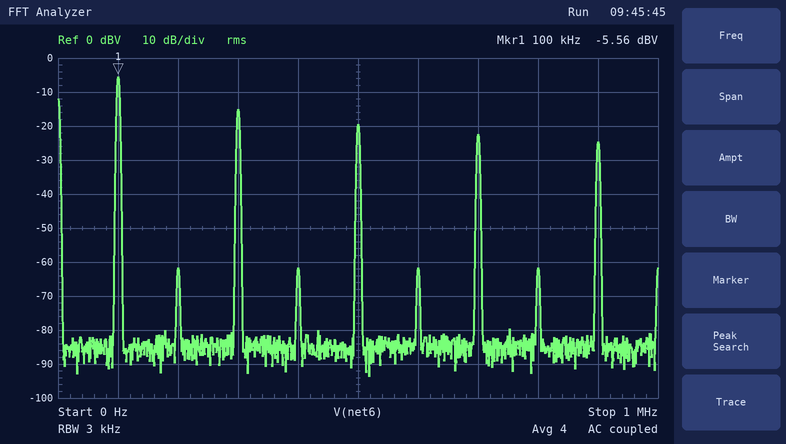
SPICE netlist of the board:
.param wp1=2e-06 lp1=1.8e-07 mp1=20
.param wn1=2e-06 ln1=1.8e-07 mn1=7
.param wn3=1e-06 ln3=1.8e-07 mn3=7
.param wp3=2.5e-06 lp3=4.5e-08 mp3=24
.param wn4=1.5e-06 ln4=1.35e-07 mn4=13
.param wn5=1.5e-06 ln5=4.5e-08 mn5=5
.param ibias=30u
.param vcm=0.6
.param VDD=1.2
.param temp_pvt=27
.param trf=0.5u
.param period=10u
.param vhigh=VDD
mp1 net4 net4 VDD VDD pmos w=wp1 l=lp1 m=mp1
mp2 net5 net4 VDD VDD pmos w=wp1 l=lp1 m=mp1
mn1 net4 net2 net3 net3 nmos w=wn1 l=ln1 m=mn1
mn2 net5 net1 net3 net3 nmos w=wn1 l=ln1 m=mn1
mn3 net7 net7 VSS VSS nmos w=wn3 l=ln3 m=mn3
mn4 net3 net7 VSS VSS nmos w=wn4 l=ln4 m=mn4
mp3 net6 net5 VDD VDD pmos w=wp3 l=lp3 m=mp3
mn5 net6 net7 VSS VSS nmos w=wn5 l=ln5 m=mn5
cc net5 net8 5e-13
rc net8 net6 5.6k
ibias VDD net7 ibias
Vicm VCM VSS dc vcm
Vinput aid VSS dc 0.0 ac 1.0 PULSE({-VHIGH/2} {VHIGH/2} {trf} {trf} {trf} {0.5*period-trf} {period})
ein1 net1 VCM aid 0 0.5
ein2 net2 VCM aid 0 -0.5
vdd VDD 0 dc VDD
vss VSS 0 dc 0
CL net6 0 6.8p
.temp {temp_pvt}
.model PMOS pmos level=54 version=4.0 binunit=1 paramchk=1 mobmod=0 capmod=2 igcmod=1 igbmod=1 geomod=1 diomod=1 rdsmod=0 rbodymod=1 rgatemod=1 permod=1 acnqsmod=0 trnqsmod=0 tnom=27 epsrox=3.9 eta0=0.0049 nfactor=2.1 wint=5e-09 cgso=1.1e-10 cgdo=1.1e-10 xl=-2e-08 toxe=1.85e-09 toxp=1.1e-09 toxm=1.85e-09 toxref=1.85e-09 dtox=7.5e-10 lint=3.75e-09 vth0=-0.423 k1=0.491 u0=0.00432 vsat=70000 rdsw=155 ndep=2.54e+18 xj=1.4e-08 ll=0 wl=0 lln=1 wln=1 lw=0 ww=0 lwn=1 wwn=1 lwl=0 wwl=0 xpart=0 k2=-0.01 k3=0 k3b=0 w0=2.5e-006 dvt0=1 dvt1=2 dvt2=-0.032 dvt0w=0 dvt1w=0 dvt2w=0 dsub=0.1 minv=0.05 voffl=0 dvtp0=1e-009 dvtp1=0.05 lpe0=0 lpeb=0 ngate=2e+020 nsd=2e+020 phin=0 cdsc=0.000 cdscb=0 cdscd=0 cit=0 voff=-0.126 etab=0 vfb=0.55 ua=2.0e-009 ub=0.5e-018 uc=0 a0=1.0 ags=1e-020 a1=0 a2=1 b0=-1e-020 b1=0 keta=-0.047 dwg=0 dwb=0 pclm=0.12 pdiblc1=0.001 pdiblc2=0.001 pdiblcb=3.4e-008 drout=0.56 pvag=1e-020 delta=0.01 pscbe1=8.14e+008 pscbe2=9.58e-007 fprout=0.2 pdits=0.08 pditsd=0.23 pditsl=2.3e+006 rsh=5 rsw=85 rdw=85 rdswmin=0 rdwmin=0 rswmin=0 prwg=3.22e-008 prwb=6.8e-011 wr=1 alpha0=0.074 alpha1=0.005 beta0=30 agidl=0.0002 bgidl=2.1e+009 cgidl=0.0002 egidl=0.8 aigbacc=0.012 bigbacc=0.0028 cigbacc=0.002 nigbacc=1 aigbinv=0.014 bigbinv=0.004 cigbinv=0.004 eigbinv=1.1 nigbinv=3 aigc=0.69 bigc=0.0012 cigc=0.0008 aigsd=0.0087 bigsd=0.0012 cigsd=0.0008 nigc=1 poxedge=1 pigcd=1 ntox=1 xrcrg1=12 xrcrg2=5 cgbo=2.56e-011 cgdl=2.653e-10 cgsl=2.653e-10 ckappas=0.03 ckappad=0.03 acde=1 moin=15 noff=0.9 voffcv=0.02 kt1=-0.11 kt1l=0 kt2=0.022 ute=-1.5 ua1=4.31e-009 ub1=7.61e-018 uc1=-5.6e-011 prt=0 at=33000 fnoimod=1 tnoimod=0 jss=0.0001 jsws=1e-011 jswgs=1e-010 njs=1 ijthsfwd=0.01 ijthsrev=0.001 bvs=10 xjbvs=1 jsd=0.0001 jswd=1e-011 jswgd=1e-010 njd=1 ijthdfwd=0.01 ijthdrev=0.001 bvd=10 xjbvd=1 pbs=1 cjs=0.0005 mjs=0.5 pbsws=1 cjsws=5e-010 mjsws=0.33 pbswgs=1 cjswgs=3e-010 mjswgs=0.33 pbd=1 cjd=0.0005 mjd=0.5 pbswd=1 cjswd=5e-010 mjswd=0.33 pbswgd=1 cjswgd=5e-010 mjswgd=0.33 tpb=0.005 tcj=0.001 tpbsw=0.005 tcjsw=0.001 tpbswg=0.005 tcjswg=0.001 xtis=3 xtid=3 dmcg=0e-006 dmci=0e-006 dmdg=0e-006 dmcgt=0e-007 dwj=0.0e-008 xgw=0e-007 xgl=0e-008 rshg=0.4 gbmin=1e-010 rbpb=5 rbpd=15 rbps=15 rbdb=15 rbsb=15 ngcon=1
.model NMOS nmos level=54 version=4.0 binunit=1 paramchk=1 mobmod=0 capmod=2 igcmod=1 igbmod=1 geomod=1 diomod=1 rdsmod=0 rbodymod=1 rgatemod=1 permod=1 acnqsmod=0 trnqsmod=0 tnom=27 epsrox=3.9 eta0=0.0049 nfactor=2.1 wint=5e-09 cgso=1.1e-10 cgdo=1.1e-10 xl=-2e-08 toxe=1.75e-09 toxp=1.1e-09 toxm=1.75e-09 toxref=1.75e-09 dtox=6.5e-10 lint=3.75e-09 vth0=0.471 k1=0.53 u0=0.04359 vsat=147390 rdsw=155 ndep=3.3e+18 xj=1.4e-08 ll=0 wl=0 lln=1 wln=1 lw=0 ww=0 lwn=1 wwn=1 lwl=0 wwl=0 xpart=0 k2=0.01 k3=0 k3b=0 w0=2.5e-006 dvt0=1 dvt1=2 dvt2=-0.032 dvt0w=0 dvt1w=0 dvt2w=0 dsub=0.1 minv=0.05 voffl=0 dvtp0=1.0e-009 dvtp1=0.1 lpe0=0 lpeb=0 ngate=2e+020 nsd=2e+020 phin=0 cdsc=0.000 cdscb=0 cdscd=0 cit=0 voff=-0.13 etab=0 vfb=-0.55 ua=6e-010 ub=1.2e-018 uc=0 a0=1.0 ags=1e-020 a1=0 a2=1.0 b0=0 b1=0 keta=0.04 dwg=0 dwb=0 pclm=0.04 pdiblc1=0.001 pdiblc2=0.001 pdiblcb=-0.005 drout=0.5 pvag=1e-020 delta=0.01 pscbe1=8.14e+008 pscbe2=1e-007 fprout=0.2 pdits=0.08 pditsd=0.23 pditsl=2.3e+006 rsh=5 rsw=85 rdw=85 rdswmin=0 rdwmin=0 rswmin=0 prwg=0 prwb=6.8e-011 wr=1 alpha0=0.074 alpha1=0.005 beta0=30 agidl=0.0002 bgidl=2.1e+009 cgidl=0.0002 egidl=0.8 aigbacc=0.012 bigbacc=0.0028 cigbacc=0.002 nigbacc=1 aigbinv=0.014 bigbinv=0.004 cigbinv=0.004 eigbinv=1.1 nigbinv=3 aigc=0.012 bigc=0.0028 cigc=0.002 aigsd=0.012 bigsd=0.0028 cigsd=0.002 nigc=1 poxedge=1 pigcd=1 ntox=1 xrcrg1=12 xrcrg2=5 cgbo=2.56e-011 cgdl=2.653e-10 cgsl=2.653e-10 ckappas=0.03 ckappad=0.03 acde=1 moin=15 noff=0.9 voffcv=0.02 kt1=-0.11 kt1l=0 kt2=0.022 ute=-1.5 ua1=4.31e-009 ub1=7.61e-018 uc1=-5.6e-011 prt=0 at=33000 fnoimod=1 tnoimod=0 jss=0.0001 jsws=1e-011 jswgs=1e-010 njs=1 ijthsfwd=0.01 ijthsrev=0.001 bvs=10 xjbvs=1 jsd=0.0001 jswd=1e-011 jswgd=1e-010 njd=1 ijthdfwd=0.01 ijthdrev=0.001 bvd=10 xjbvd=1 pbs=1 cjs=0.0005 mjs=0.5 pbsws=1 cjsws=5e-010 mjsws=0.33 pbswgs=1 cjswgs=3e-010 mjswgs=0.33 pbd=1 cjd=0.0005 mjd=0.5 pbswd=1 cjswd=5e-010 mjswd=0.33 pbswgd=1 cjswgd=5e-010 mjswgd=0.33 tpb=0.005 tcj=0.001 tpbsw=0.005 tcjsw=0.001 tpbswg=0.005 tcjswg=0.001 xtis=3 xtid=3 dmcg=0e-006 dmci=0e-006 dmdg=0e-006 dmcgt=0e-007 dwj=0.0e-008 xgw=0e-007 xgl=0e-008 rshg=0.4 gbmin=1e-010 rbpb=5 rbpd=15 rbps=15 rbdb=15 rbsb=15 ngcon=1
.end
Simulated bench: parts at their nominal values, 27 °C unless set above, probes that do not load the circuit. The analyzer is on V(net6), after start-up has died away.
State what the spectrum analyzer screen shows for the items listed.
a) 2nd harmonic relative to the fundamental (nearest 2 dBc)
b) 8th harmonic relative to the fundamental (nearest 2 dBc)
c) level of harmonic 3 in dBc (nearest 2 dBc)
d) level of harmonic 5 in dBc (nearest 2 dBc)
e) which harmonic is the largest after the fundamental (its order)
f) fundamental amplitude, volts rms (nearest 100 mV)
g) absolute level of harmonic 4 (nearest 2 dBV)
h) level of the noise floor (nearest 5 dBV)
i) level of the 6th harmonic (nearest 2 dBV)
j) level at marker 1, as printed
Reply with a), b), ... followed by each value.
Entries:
a) -56 dBc
b) -56 dBc
c) -10 dBc
d) -14 dBc
e) 3
f) 500 mV
g) -62 dBV
h) -85 dBV
i) -62 dBV
j) -5.56 dBV
